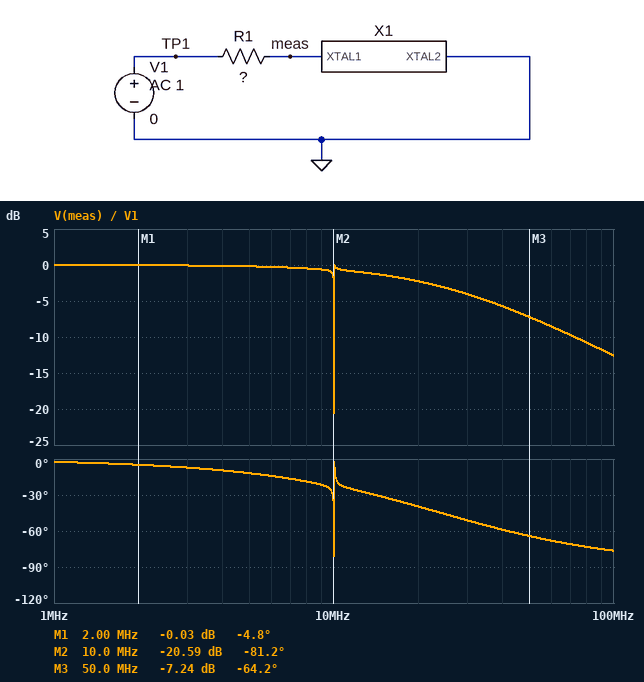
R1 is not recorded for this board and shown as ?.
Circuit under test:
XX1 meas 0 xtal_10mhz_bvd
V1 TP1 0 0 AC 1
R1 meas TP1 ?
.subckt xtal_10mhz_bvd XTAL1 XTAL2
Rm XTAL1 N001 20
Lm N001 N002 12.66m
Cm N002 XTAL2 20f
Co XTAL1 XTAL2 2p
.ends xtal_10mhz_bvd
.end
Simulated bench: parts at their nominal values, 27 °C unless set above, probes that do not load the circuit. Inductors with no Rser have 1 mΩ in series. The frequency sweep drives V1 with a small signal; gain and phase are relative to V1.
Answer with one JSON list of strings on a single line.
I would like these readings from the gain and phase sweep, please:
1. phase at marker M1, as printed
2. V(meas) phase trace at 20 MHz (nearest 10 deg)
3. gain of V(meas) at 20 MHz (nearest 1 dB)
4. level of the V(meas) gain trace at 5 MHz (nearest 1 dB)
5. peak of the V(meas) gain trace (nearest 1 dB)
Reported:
["-4.8 deg", "-40 deg", "-2 dB", "0 dB", "0 dB"]
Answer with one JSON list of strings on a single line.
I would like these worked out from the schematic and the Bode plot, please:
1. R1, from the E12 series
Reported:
["3.3 kΩ"]
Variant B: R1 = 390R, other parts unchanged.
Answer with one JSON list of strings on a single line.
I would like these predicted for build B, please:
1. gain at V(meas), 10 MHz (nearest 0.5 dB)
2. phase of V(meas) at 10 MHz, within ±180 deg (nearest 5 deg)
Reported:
["-4.5 dB", "-50 deg"]
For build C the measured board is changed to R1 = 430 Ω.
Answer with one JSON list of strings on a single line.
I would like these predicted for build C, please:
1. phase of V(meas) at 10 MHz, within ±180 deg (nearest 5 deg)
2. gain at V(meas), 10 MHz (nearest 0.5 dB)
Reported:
["-50 deg", "-5.0 dB"]
